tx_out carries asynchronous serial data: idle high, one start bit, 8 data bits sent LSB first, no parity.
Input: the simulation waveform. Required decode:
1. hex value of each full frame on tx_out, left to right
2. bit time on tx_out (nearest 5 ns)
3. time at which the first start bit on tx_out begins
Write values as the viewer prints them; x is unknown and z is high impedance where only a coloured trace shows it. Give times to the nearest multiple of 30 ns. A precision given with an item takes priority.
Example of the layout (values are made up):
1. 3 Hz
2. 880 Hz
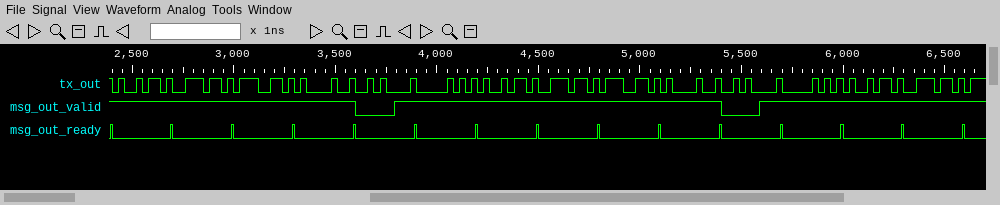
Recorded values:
1. 69, 6E, 67, 21, 0A, 50, 69, 6E, 67, 21, 0A, 50, 69, 6E
2. 30 ns
3. 2400 ns
